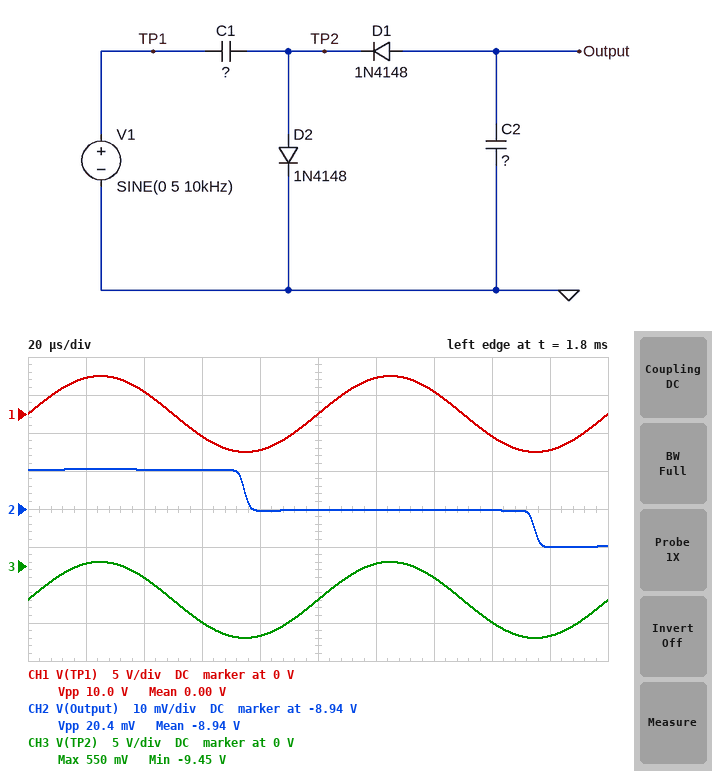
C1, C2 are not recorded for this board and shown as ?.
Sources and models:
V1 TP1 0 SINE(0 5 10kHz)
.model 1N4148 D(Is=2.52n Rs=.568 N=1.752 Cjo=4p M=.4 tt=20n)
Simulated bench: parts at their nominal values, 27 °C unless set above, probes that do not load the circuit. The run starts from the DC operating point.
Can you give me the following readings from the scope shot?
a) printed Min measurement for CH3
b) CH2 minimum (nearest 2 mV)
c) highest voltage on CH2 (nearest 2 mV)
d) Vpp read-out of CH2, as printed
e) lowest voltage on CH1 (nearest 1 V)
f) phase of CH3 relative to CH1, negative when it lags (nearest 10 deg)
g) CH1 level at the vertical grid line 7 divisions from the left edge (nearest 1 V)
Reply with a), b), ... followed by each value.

a) -9.45 V
b) -8.950 V
c) -8.930 V
d) 20.4 mV
e) -5 V
f) 0 deg
g) 3 V
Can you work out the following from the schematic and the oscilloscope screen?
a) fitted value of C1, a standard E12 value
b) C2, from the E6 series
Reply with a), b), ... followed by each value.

a) 47 nF
b) 100 nF
